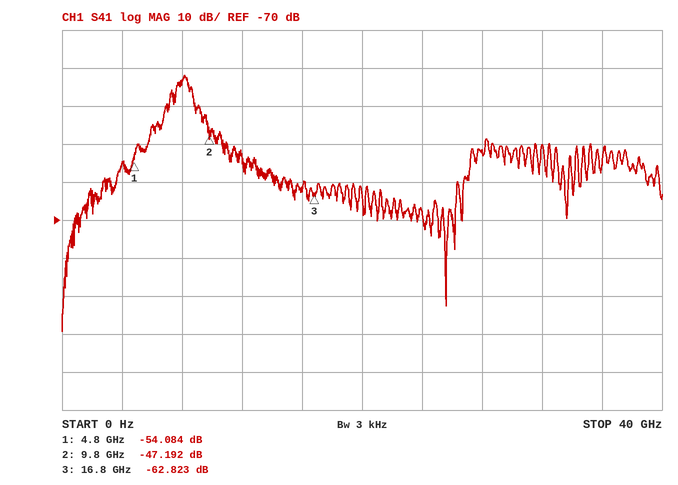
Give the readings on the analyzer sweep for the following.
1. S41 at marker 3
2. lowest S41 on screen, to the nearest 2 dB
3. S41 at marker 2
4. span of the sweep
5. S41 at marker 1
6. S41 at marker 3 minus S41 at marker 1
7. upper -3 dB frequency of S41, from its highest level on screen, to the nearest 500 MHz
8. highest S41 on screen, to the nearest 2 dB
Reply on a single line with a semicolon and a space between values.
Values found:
-62.823 dB; -100 dB; -47.192 dB; 40 GHz; -54.084 dB; -8.739 dB; 8.5 GHz; -32 dB
